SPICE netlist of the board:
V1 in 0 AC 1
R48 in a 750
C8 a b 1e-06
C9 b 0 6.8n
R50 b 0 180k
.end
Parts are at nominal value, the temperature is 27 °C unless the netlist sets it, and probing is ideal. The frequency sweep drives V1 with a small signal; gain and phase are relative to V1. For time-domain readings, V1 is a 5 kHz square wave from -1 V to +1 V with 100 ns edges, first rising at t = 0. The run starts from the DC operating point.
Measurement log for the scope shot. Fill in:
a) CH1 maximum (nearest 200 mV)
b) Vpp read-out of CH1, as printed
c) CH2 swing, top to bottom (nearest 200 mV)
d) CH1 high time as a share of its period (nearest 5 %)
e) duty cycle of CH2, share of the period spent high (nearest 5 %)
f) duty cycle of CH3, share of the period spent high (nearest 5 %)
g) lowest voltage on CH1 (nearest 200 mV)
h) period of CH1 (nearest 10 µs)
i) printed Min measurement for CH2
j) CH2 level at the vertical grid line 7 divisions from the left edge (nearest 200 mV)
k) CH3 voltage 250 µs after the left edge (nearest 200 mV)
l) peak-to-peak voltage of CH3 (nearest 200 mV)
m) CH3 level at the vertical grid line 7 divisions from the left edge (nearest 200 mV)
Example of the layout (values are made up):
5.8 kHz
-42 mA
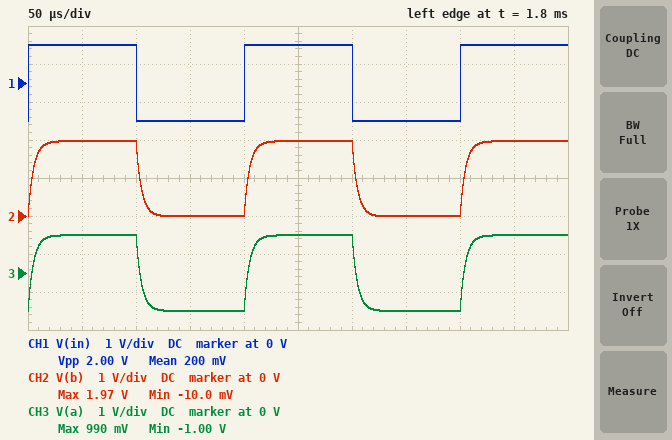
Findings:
1.0 V
2.00 V
2.0 V
50 %
50 %
50 %
-1.0 V
200 µs
-10.0 mV
0 V
1.0 V
2.0 V
-1.0 V
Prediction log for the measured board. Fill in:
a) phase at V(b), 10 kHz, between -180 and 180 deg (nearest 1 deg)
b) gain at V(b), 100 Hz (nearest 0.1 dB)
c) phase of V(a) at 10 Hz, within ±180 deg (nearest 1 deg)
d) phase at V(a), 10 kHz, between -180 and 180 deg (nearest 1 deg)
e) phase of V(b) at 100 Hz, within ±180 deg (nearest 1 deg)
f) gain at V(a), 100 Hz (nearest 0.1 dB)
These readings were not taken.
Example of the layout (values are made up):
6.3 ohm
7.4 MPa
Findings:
-18 deg
-0.1 dB
0 deg
-18 deg
0 deg
0 dB
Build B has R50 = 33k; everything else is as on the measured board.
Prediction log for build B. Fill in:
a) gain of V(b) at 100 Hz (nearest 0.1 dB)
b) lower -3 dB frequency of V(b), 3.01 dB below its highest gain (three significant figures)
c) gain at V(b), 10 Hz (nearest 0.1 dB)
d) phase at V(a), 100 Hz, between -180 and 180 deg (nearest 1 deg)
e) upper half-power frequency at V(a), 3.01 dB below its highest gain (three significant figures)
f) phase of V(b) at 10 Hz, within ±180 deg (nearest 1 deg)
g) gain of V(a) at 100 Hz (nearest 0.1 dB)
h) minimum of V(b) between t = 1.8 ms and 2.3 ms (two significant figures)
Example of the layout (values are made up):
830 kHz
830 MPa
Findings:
-0.3 dB
4.68 Hz
-1.1 dB
0 deg
30.7 kHz
25 deg
-0.2 dB
-61 mV
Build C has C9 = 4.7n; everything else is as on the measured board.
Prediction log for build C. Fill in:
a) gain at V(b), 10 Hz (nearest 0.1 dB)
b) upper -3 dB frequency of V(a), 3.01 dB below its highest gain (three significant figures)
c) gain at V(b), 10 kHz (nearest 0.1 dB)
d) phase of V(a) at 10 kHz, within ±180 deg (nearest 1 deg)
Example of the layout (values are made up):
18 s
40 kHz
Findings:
-0.1 dB
45.2 kHz
-0.3 dB
-12 deg
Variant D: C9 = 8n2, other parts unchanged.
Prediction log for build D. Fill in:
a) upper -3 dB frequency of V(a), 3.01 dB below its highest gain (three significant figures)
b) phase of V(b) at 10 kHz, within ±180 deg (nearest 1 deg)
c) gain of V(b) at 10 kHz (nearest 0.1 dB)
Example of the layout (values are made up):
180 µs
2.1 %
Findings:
26.0 kHz
-21 deg
-0.7 dB
